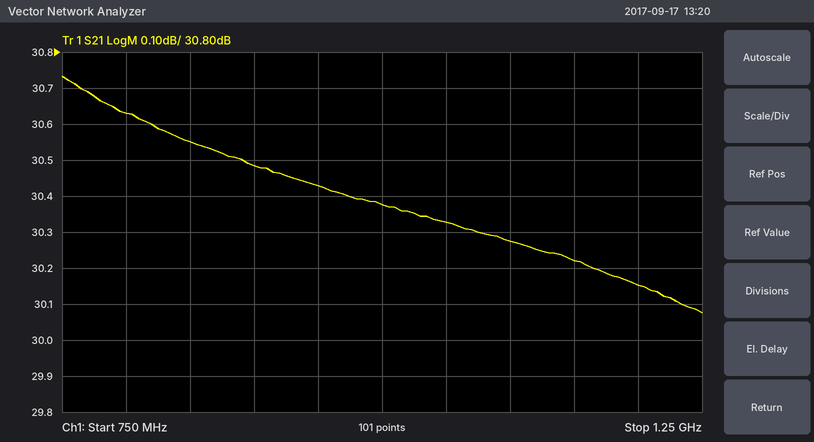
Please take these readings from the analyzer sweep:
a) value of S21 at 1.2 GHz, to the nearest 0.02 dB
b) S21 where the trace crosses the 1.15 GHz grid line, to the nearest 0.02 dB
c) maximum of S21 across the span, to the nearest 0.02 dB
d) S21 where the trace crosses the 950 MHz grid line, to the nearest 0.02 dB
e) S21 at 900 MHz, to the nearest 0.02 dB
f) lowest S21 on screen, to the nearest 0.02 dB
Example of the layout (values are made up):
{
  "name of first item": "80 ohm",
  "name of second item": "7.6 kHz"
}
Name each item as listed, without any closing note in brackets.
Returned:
{
  "value of S21 at 1.2 GHz, to the nearest 0.02 dB": "30.16 dB",
  "S21 where the trace crosses the 1.15 GHz grid line, to the nearest 0.02 dB": "30.22 dB",
  "maximum of S21 across the span, to the nearest 0.02 dB": "30.74 dB",
  "S21 where the trace crosses the 950 MHz grid line, to the nearest 0.02 dB": "30.42 dB",
  "S21 at 900 MHz, to the nearest 0.02 dB": "30.48 dB",
  "lowest S21 on screen, to the nearest 0.02 dB": "30.08 dB"
}
